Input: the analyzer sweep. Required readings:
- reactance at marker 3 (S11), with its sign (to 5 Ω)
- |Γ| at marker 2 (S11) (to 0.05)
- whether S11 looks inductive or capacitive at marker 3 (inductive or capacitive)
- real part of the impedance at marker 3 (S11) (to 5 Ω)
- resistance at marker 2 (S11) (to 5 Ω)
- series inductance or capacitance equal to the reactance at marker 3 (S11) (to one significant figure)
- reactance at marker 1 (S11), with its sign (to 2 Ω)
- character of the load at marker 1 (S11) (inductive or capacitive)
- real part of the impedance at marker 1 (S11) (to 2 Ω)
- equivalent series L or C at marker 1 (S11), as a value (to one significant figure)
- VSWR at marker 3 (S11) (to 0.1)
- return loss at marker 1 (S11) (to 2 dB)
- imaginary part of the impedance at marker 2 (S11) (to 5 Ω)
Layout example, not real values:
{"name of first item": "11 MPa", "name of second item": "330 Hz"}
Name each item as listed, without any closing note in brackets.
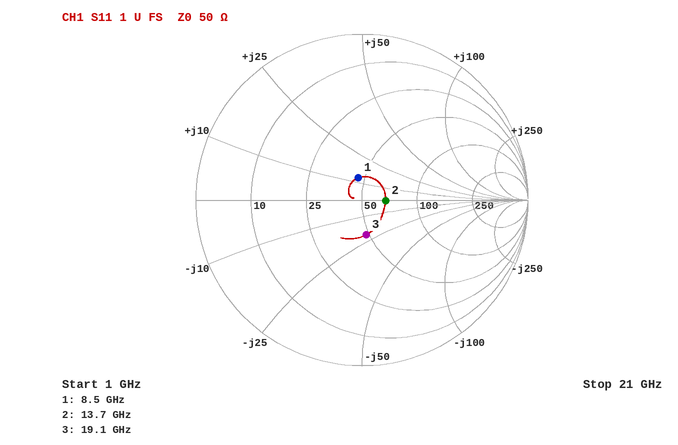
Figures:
{"reactance at marker 3 (S11), with its sign": "-20 Ω", "|Γ| at marker 2 (S11)": "0.15", "whether S11 looks inductive or capacitive at marker 3": "capacitive", "real part of the impedance at marker 3 (S11)": "50 Ω", "resistance at marker 2 (S11)": "65 Ω", "series inductance or capacitance equal to the reactance at marker 3 (S11)": "400 fF", "reactance at marker 1 (S11), with its sign": "+12 Ω", "character of the load at marker 1 (S11)": "inductive", "real part of the impedance at marker 1 (S11)": "46 Ω", "equivalent series L or C at marker 1 (S11), as a value": "200 pH", "VSWR at marker 3 (S11)": "1.5", "return loss at marker 1 (S11)": "18 dB", "imaginary part of the impedance at marker 2 (S11)": "0 Ω"}
